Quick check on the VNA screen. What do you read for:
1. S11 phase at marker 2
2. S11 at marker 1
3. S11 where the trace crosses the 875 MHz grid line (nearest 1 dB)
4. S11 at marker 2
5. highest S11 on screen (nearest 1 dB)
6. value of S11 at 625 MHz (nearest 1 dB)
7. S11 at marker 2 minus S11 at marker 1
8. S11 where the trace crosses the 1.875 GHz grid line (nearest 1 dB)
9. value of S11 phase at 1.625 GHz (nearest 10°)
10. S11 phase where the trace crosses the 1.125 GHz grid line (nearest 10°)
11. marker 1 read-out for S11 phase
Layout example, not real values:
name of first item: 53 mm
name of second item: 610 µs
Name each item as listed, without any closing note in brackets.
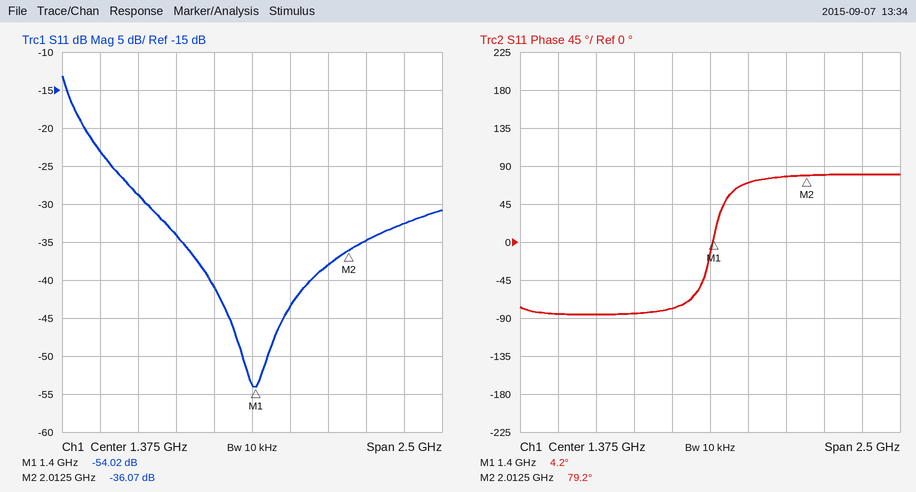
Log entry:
S11 phase at marker 2: 79.2°
S11 at marker 1: -54.02 dB
S11 where the trace crosses the 875 MHz grid line: -34 dB
S11 at marker 2: -36.07 dB
highest S11 on screen: -13 dB
value of S11 at 625 MHz: -29 dB
S11 at marker 2 minus S11 at marker 1: 17.95 dB
S11 where the trace crosses the 1.875 GHz grid line: -38 dB
value of S11 phase at 1.625 GHz: 70°
S11 phase where the trace crosses the 1.125 GHz grid line: -80°
marker 1 read-out for S11 phase: 4.2°
